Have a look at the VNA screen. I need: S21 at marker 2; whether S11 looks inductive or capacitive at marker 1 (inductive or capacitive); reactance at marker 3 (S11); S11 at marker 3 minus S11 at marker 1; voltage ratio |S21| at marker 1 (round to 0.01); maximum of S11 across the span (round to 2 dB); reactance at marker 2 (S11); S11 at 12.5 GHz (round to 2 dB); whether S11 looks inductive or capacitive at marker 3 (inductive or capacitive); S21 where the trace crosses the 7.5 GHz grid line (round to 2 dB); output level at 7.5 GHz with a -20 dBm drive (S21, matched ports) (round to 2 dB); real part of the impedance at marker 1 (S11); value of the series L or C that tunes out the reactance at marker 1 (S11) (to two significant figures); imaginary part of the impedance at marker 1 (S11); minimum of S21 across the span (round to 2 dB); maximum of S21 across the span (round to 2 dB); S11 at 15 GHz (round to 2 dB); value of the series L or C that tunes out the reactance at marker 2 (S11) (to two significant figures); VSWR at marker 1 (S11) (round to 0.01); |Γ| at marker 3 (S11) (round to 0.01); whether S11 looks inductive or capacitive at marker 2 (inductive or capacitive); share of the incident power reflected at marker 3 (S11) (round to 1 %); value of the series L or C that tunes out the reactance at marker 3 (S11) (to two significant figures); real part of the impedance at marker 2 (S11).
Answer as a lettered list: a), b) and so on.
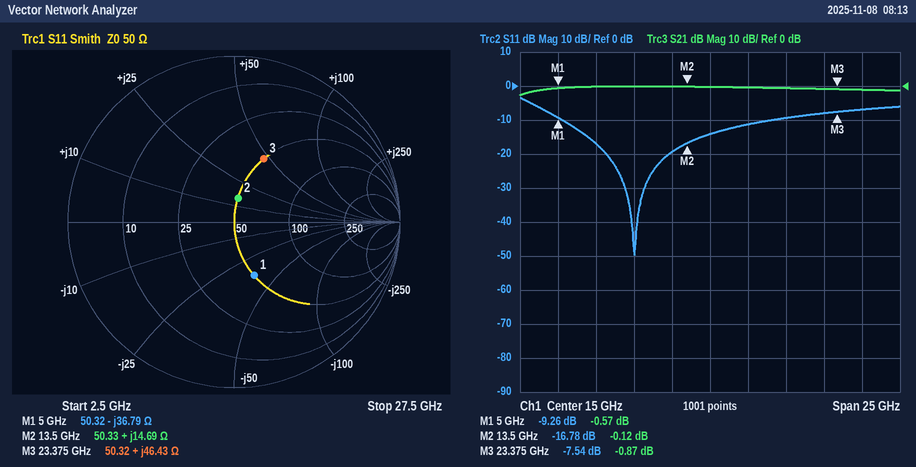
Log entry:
a) -0.12 dB
b) capacitive
c) +46.43 Ω
d) 1.72 dB
e) 0.94
f) -4 dB
g) +14.69 Ω
h) -20 dB
i) inductive
j) 0 dB
k) -20 dBm
l) 50.32 Ω
m) 1.2 nH
n) -36.79 Ω
o) -2 dB
p) 0 dB
q) -14 dB
r) 800 fF
s) 2.05
t) 0.42
u) inductive
v) 18 %
w) 150 fF
x) 50.33 Ω
